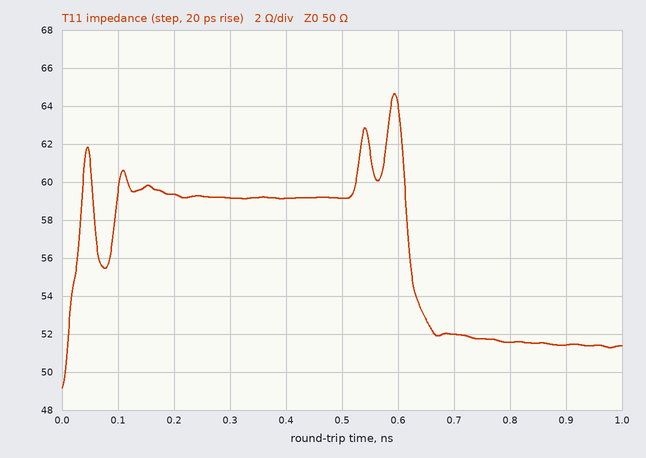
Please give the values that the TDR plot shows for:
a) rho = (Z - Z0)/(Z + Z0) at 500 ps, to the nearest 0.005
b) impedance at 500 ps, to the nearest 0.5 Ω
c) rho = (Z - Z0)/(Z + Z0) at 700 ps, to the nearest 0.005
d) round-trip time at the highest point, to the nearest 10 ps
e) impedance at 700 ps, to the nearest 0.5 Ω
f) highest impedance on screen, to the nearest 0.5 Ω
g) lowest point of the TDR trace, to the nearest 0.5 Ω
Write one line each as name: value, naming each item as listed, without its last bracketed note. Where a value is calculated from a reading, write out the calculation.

rho = (Z - Z0)/(Z + Z0) at 500 ps, to the nearest 0.005: (59 − 50)/(59 + 50) ≈ +0.0826, so +0.085 to the nearest 0.005
impedance at 500 ps, to the nearest 0.5 Ω: 59.0 Ω
rho = (Z - Z0)/(Z + Z0) at 700 ps, to the nearest 0.005: (52 − 50)/(52 + 50) ≈ +0.020
round-trip time at the highest point, to the nearest 10 ps: 590 ps
impedance at 700 ps, to the nearest 0.5 Ω: 52.0 Ω
highest impedance on screen, to the nearest 0.5 Ω: 64.5 Ω
lowest point of the TDR trace, to the nearest 0.5 Ω: 49.0 Ω
